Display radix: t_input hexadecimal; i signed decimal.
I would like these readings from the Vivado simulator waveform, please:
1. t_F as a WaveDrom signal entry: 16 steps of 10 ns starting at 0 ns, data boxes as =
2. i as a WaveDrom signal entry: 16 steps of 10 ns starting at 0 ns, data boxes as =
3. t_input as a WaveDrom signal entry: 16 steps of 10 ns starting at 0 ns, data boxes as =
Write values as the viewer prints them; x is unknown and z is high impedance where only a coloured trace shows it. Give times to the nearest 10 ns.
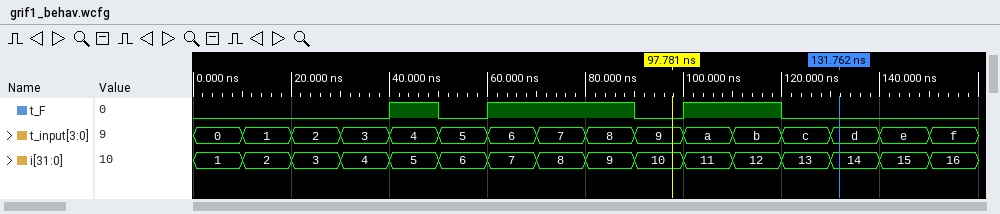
{name: 't_F', wave: '0...101..01.0...'}
{name: 'i', wave: '================', data: '1 2 3 4 5 6 7 8 9 10 11 12 13 14 15 16'}
{name: 't_input', wave: '================', data: '0 1 2 3 4 5 6 7 8 9 a b c d e f'}
